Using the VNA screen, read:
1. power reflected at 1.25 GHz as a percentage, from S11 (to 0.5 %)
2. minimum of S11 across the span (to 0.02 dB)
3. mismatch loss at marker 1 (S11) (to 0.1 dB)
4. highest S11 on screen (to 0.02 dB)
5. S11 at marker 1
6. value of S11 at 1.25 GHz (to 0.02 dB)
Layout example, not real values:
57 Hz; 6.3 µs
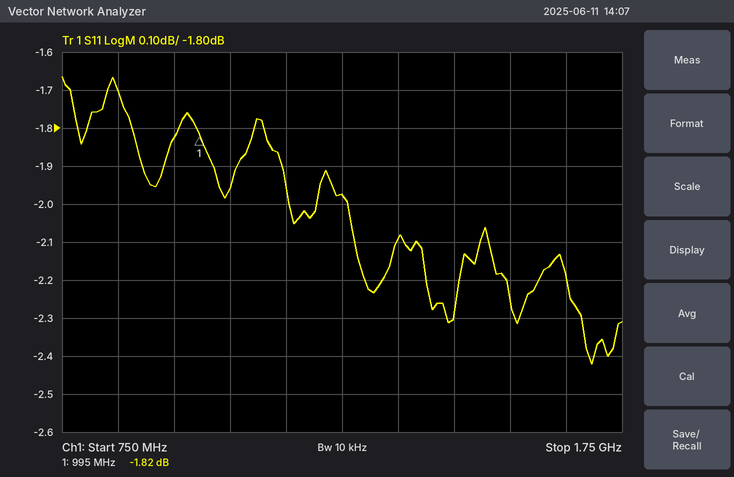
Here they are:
63.5 %; -2.42 dB; 4.7 dB; -1.66 dB; -1.82 dB; -1.98 dB
